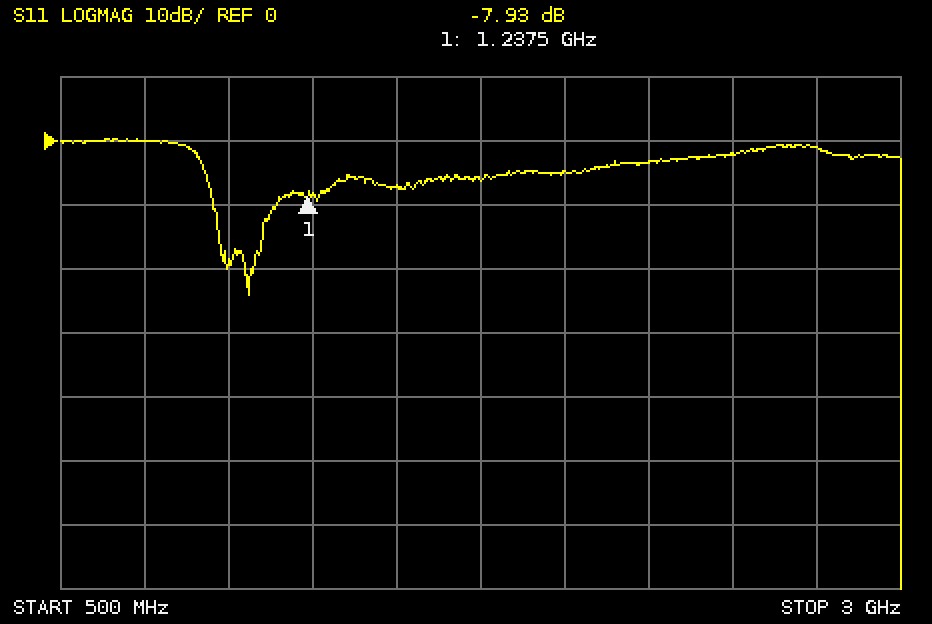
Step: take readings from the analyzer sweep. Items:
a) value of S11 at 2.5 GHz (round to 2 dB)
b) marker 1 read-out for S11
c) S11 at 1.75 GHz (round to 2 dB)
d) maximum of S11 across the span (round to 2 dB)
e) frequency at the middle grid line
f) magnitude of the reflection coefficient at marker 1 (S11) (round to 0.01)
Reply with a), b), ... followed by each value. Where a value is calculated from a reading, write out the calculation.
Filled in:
a) -2 dB
b) -7.93 dB
c) -6 dB
d) 0 dB
e) 1.75 GHz
f) 10^(-7.93/20) ≈ 0.40
